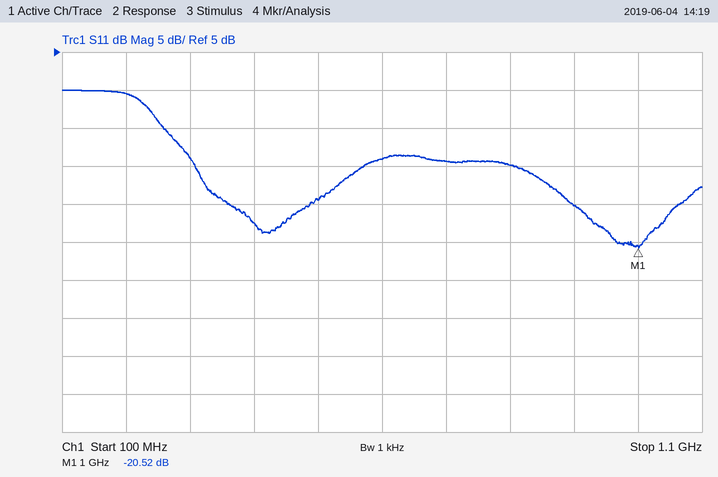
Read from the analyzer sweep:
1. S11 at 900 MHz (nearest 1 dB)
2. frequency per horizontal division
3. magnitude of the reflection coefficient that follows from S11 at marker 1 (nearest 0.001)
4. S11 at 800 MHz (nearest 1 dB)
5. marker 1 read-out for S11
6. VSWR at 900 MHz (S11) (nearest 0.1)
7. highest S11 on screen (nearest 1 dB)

-15 dB
100 MHz
0.094
-10 dB
-20.52 dB
1.4
0 dB
